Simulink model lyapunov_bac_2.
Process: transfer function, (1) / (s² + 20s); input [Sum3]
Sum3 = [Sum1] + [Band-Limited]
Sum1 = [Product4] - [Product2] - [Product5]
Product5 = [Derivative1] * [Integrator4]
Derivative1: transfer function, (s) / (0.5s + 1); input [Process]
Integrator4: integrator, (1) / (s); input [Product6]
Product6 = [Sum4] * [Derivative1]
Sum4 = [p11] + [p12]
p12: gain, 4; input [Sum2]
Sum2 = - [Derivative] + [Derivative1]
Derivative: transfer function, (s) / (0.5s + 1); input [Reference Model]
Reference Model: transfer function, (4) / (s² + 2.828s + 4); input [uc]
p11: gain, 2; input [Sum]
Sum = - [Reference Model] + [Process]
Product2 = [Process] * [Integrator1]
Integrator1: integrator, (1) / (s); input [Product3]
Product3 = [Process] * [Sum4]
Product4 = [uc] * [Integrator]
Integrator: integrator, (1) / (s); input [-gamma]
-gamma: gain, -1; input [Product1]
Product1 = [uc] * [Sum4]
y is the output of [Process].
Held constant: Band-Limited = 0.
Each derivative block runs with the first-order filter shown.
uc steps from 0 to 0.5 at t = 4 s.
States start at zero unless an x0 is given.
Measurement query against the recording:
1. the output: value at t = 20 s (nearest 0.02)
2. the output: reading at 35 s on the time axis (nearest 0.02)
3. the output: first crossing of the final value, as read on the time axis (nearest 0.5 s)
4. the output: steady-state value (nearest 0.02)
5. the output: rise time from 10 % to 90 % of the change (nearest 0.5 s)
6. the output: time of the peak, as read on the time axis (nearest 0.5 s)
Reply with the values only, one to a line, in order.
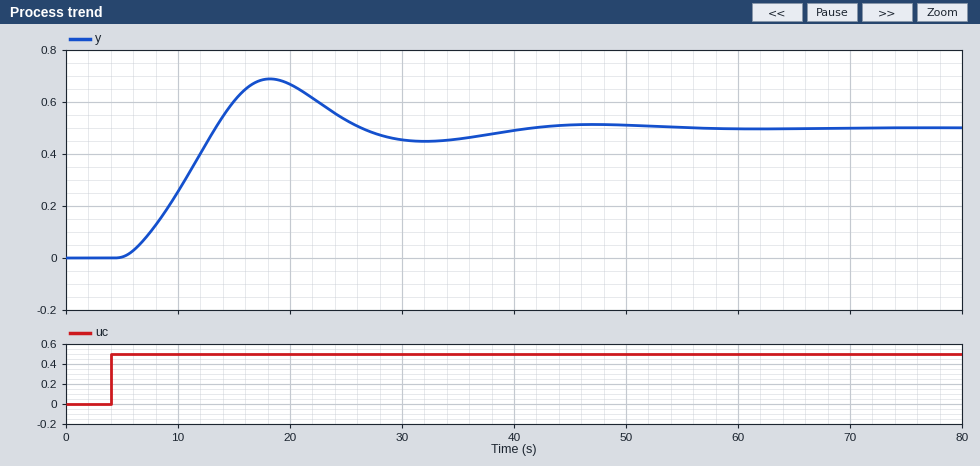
0.66
0.46
13.5 s
0.50
6.0 s
18.0 s
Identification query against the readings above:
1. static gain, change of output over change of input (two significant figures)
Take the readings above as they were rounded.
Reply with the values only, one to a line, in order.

1.0
